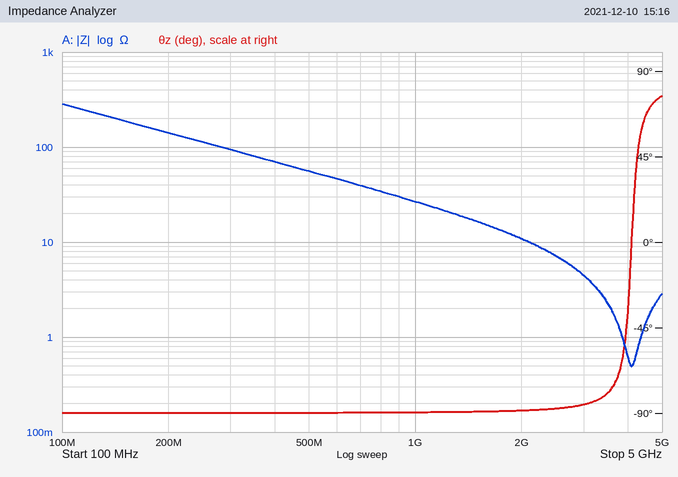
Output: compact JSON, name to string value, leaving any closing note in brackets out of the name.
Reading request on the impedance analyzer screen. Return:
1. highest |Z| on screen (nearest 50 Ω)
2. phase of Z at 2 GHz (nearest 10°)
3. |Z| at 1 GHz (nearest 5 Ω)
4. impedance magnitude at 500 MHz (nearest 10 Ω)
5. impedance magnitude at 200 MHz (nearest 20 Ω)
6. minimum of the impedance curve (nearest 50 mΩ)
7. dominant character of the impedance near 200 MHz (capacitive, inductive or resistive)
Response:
{"highest |Z| on screen": "300 Ω", "phase of Z at 2 GHz": "-90°", "|Z| at 1 GHz": "25 Ω", "impedance magnitude at 500 MHz": "60 Ω", "impedance magnitude at 200 MHz": "140 Ω", "minimum of the impedance curve": "500 mΩ", "dominant character of the impedance near 200 MHz": "capacitive"}
